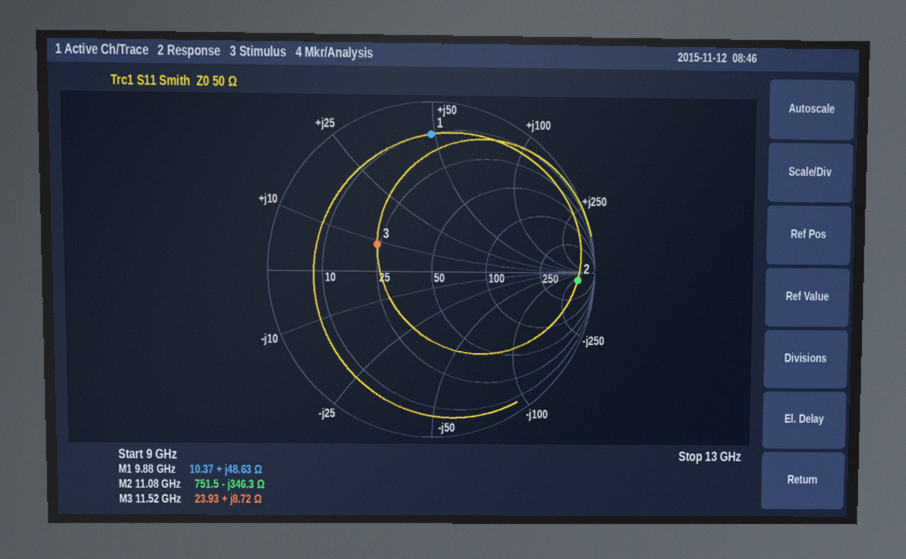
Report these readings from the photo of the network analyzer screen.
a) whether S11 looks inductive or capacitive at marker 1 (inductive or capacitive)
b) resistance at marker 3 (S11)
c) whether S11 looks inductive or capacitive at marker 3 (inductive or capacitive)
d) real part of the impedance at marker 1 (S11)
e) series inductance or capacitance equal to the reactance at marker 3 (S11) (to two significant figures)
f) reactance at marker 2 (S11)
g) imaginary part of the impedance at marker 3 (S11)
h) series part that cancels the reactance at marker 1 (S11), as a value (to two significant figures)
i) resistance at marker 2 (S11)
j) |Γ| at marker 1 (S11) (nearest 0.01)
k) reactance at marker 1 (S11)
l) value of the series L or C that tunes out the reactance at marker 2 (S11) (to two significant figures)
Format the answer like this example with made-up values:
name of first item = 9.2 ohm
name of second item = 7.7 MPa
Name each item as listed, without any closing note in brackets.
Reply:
whether S11 looks inductive or capacitive at marker 1 = inductive
resistance at marker 3 = 23.93 Ω
whether S11 looks inductive or capacitive at marker 3 = inductive
real part of the impedance at marker 1 = 10.37 Ω
series inductance or capacitance equal to the reactance at marker 3 (S11) = 120 pH
reactance at marker 2 = -346.3 Ω
imaginary part of the impedance at marker 3 = +8.72 Ω
series part that cancels the reactance at marker 1 (S11), as a value = 330 fF
resistance at marker 2 = 751.5 Ω
|Γ| at marker 1 (S11) = 0.81
reactance at marker 1 = +48.63 Ω
value of the series L or C that tunes out the reactance at marker 2 (S11) = 5.0 nH
